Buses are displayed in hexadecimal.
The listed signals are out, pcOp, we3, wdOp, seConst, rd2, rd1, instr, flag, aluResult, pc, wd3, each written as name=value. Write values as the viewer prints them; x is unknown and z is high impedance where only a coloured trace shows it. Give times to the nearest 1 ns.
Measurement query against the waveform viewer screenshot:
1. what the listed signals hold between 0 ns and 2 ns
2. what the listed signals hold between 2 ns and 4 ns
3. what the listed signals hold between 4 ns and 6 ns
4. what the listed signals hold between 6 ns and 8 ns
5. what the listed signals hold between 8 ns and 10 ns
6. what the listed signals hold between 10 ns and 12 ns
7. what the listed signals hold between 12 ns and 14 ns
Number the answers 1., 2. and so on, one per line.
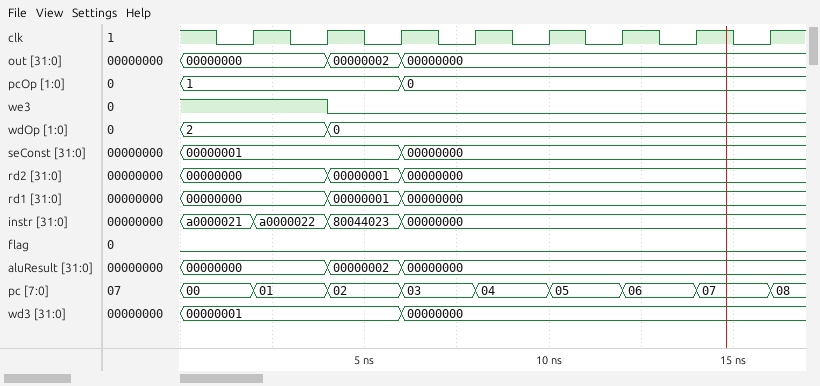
1. out=00000000, pcOp=1, we3=1, wdOp=2, seConst=00000001, rd2=00000000, rd1=00000000, instr=a0000021, flag=0, aluResult=00000000, pc=00, wd3=00000001
2. out=00000000, pcOp=1, we3=1, wdOp=2, seConst=00000001, rd2=00000000, rd1=00000000, instr=a0000022, flag=0, aluResult=00000000, pc=01, wd3=00000001
3. out=00000002, pcOp=1, we3=0, wdOp=0, seConst=00000001, rd2=00000001, rd1=00000001, instr=80044023, flag=0, aluResult=00000002, pc=02, wd3=00000001
4. out=00000000, pcOp=0, we3=0, wdOp=0, seConst=00000000, rd2=00000000, rd1=00000000, instr=00000000, flag=0, aluResult=00000000, pc=03, wd3=00000000
5. out=00000000, pcOp=0, we3=0, wdOp=0, seConst=00000000, rd2=00000000, rd1=00000000, instr=00000000, flag=0, aluResult=00000000, pc=04, wd3=00000000
6. out=00000000, pcOp=0, we3=0, wdOp=0, seConst=00000000, rd2=00000000, rd1=00000000, instr=00000000, flag=0, aluResult=00000000, pc=05, wd3=00000000
7. out=00000000, pcOp=0, we3=0, wdOp=0, seConst=00000000, rd2=00000000, rd1=00000000, instr=00000000, flag=0, aluResult=00000000, pc=06, wd3=00000000
